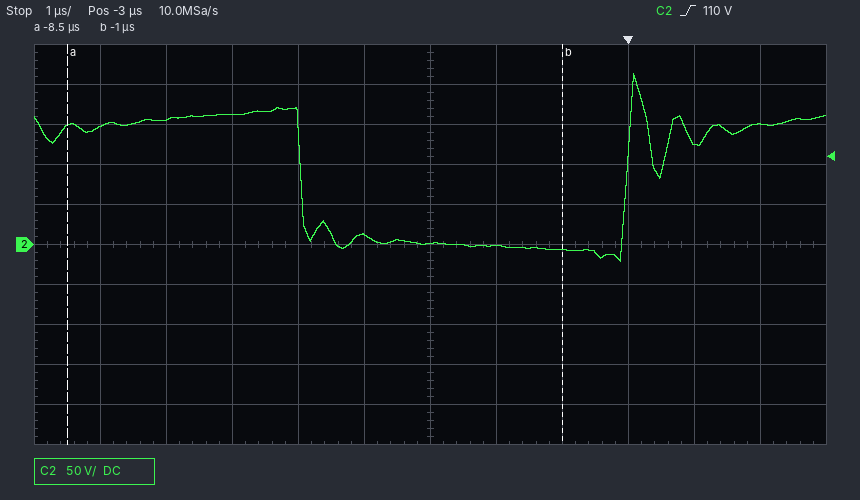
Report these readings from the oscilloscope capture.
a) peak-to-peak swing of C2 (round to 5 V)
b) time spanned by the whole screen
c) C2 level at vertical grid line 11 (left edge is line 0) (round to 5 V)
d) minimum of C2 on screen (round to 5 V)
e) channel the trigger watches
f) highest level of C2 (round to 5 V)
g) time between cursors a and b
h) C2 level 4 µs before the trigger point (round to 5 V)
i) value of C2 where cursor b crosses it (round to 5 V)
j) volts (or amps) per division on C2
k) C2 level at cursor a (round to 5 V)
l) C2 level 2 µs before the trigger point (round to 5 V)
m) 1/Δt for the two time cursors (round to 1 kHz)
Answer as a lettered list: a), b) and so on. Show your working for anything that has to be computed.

a) 215 V − (-20 V) = 235 V
b) 12 µs
c) 150 V
d) -20 V
e) C2
f) 215 V
g) -1 µs − (-8.5 µs) = 7.5 µs
h) 10 V
i) -5 V
j) 50 V
k) 150 V
l) 0 V
m) 1 / 7.5 µs ≈ 133 kHz
